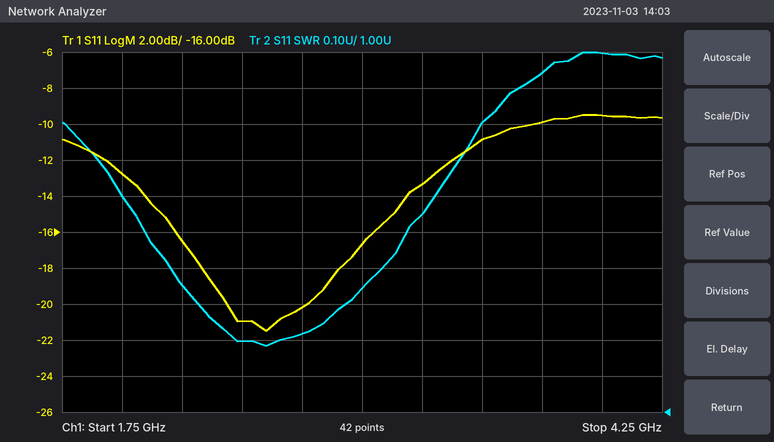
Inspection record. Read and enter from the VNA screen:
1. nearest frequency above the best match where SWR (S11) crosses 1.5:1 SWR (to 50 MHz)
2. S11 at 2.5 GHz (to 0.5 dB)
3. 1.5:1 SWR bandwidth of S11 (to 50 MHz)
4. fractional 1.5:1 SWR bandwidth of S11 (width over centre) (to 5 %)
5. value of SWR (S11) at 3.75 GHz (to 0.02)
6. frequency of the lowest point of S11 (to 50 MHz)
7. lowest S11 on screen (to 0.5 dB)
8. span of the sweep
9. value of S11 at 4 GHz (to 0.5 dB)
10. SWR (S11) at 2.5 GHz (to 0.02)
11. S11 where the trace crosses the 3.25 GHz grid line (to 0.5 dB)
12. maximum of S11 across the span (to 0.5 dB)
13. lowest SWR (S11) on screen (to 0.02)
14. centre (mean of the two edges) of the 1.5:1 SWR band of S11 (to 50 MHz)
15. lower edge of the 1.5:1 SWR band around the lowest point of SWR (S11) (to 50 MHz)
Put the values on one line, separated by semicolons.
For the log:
3.20 GHz; -21.0 dB; 1.10 GHz; 40 %; 1.94; 2.60 GHz; -21.5 dB; 2.5 GHz; -9.5 dB; 1.20; -13.5 dB; -9.5 dB; 1.18; 2.65 GHz; 2.10 GHz
